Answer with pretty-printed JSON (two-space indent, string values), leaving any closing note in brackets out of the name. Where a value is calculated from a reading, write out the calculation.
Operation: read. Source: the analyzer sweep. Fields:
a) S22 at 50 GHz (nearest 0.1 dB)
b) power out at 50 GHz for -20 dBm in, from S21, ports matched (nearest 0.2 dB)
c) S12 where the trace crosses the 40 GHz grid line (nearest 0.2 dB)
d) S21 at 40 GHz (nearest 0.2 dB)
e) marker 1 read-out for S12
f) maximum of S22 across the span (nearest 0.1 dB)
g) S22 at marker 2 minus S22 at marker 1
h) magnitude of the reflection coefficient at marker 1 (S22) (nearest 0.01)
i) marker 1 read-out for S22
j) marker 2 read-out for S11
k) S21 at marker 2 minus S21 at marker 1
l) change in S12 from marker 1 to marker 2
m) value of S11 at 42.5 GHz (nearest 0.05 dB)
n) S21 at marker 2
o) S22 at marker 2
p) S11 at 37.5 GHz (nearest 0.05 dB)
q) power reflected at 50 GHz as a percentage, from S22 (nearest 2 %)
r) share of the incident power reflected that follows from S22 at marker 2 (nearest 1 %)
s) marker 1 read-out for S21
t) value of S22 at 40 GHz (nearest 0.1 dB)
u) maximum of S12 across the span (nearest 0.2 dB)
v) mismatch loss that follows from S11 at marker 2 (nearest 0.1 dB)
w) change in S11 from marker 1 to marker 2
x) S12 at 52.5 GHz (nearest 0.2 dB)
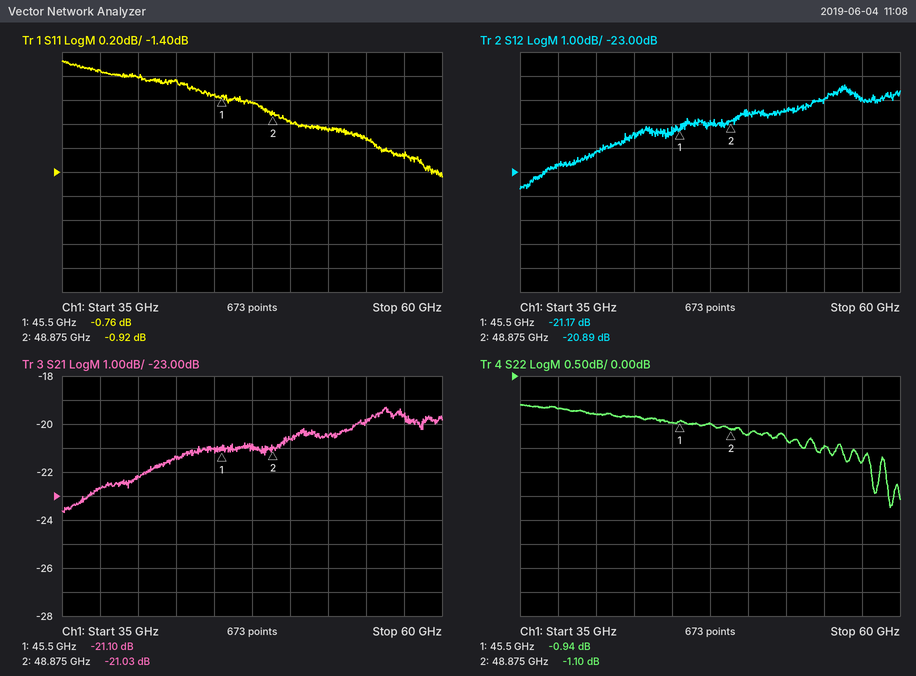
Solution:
{
  "S22 at 50 GHz": "-1.2 dB",
  "power out at 50 GHz for -20 dBm in, from S21, ports matched": "-20 dBm + (-20.6 dB) = -40.6 dBm",
  "S12 where the trace crosses the 40 GHz grid line": "-22.2 dB",
  "S21 at 40 GHz": "-22.2 dB",
  "marker 1 read-out for S12": "-21.17 dB",
  "maximum of S22 across the span": "-0.6 dB",
  "S22 at marker 2 minus S22 at marker 1": "-1.1 − (-0.94) = -0.16 dB",
  "magnitude of the reflection coefficient at marker 1 (S22)": "10^(-0.94/20) ≈ 0.90",
  "marker 1 read-out for S22": "-0.94 dB",
  "marker 2 read-out for S11": "-0.92 dB",
  "S21 at marker 2 minus S21 at marker 1": "-21.03 − (-21.1) = 0.07 dB",
  "change in S12 from marker 1 to marker 2": "-20.89 − (-21.17) = 0.28 dB",
  "value of S11 at 42.5 GHz": "-0.65 dB",
  "S21 at marker 2": "-21.03 dB",
  "S22 at marker 2": "-1.10 dB",
  "S11 at 37.5 GHz": "-0.55 dB",
  "power reflected at 50 GHz as a percentage, from S22": "10^(-1.2/10) ≈ 76 %",
  "share of the incident power reflected that follows from S22 at marker 2": "10^(-1.1/10) ≈ 78 %",
  "marker 1 read-out for S21": "-21.10 dB",
  "value of S22 at 40 GHz": "-0.8 dB",
  "maximum of S12 across the span": "-19.4 dB",
  "mismatch loss that follows from S11 at marker 2": "−10 log10(1 − 10^(-0.92/10)) ≈ 7.2 dB",
  "change in S11 from marker 1 to marker 2": "-0.92 − (-0.76) = -0.16 dB",
  "S12 at 52.5 GHz": "-20.4 dB"
}
